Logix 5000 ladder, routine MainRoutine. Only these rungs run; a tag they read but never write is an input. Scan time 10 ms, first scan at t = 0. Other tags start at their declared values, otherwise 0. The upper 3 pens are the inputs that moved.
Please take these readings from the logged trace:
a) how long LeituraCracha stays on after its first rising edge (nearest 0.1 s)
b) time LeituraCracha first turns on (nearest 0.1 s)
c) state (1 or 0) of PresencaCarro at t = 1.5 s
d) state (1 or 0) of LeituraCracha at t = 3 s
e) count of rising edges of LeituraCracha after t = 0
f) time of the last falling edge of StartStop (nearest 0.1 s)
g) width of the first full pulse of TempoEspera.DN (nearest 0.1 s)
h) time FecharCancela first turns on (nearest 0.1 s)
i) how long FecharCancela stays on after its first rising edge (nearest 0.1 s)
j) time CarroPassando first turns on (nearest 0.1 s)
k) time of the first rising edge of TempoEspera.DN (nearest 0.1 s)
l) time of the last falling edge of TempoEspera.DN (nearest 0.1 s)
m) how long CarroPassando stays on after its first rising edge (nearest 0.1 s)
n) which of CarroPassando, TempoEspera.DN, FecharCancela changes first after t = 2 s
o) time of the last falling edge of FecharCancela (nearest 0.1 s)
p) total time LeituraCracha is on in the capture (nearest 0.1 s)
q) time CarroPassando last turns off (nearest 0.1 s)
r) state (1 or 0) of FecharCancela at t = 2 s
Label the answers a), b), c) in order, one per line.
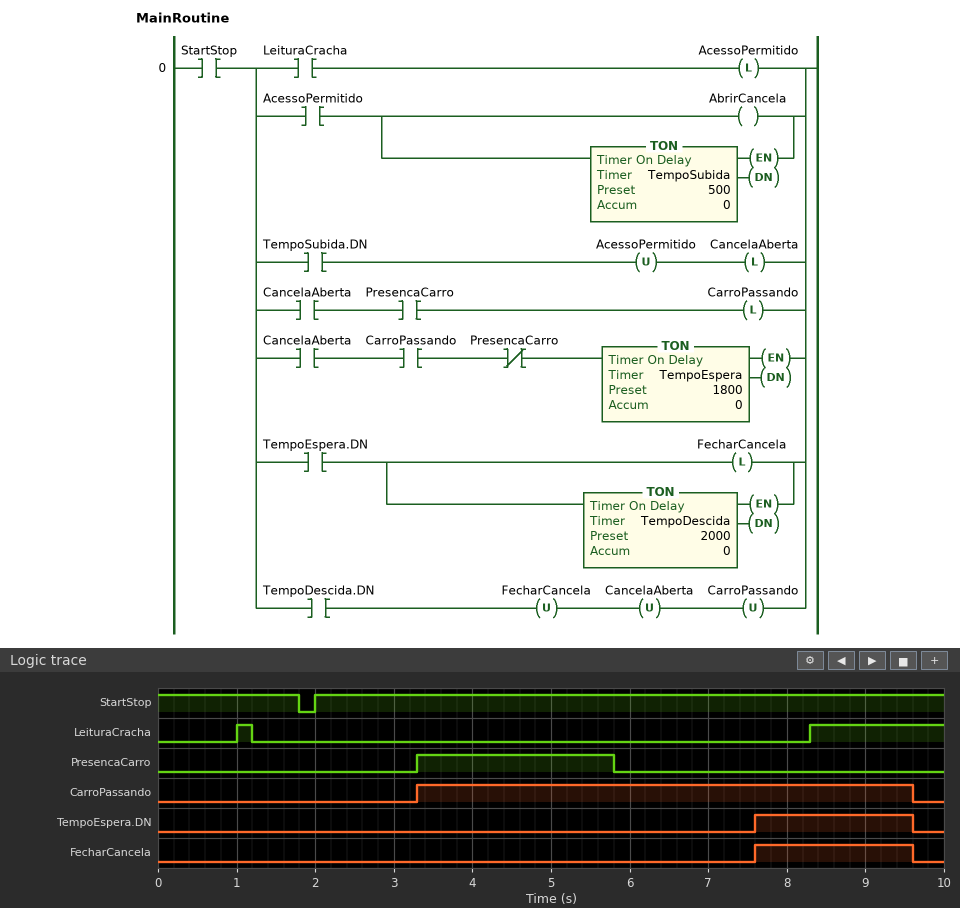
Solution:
a) 0.2 s
b) 1.0 s
c) 0
d) 0
e) 2
f) 1.8 s
g) 2.0 s
h) 7.6 s
i) 2.0 s
j) 3.3 s
k) 7.6 s
l) 9.6 s
m) 6.3 s
n) CarroPassando
o) 9.6 s
p) 1.9 s
q) 9.6 s
r) 0
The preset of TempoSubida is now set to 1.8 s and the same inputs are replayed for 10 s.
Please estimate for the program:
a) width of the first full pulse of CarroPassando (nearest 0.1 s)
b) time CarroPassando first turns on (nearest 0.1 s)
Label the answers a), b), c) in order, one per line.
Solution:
a) 5.8 s
b) 3.8 s
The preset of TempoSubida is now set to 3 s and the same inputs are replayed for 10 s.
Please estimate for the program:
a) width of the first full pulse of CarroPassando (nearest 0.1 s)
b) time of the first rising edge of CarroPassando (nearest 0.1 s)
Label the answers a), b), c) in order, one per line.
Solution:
a) 4.6 s
b) 5.0 s
